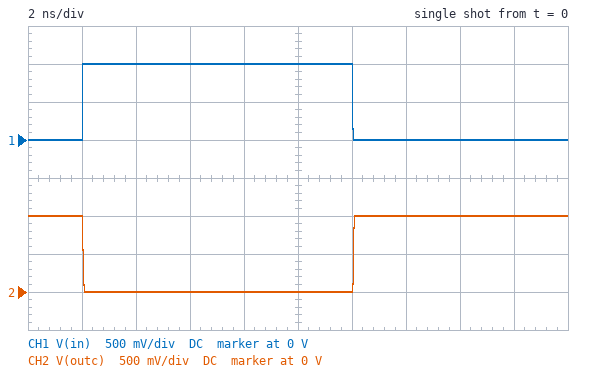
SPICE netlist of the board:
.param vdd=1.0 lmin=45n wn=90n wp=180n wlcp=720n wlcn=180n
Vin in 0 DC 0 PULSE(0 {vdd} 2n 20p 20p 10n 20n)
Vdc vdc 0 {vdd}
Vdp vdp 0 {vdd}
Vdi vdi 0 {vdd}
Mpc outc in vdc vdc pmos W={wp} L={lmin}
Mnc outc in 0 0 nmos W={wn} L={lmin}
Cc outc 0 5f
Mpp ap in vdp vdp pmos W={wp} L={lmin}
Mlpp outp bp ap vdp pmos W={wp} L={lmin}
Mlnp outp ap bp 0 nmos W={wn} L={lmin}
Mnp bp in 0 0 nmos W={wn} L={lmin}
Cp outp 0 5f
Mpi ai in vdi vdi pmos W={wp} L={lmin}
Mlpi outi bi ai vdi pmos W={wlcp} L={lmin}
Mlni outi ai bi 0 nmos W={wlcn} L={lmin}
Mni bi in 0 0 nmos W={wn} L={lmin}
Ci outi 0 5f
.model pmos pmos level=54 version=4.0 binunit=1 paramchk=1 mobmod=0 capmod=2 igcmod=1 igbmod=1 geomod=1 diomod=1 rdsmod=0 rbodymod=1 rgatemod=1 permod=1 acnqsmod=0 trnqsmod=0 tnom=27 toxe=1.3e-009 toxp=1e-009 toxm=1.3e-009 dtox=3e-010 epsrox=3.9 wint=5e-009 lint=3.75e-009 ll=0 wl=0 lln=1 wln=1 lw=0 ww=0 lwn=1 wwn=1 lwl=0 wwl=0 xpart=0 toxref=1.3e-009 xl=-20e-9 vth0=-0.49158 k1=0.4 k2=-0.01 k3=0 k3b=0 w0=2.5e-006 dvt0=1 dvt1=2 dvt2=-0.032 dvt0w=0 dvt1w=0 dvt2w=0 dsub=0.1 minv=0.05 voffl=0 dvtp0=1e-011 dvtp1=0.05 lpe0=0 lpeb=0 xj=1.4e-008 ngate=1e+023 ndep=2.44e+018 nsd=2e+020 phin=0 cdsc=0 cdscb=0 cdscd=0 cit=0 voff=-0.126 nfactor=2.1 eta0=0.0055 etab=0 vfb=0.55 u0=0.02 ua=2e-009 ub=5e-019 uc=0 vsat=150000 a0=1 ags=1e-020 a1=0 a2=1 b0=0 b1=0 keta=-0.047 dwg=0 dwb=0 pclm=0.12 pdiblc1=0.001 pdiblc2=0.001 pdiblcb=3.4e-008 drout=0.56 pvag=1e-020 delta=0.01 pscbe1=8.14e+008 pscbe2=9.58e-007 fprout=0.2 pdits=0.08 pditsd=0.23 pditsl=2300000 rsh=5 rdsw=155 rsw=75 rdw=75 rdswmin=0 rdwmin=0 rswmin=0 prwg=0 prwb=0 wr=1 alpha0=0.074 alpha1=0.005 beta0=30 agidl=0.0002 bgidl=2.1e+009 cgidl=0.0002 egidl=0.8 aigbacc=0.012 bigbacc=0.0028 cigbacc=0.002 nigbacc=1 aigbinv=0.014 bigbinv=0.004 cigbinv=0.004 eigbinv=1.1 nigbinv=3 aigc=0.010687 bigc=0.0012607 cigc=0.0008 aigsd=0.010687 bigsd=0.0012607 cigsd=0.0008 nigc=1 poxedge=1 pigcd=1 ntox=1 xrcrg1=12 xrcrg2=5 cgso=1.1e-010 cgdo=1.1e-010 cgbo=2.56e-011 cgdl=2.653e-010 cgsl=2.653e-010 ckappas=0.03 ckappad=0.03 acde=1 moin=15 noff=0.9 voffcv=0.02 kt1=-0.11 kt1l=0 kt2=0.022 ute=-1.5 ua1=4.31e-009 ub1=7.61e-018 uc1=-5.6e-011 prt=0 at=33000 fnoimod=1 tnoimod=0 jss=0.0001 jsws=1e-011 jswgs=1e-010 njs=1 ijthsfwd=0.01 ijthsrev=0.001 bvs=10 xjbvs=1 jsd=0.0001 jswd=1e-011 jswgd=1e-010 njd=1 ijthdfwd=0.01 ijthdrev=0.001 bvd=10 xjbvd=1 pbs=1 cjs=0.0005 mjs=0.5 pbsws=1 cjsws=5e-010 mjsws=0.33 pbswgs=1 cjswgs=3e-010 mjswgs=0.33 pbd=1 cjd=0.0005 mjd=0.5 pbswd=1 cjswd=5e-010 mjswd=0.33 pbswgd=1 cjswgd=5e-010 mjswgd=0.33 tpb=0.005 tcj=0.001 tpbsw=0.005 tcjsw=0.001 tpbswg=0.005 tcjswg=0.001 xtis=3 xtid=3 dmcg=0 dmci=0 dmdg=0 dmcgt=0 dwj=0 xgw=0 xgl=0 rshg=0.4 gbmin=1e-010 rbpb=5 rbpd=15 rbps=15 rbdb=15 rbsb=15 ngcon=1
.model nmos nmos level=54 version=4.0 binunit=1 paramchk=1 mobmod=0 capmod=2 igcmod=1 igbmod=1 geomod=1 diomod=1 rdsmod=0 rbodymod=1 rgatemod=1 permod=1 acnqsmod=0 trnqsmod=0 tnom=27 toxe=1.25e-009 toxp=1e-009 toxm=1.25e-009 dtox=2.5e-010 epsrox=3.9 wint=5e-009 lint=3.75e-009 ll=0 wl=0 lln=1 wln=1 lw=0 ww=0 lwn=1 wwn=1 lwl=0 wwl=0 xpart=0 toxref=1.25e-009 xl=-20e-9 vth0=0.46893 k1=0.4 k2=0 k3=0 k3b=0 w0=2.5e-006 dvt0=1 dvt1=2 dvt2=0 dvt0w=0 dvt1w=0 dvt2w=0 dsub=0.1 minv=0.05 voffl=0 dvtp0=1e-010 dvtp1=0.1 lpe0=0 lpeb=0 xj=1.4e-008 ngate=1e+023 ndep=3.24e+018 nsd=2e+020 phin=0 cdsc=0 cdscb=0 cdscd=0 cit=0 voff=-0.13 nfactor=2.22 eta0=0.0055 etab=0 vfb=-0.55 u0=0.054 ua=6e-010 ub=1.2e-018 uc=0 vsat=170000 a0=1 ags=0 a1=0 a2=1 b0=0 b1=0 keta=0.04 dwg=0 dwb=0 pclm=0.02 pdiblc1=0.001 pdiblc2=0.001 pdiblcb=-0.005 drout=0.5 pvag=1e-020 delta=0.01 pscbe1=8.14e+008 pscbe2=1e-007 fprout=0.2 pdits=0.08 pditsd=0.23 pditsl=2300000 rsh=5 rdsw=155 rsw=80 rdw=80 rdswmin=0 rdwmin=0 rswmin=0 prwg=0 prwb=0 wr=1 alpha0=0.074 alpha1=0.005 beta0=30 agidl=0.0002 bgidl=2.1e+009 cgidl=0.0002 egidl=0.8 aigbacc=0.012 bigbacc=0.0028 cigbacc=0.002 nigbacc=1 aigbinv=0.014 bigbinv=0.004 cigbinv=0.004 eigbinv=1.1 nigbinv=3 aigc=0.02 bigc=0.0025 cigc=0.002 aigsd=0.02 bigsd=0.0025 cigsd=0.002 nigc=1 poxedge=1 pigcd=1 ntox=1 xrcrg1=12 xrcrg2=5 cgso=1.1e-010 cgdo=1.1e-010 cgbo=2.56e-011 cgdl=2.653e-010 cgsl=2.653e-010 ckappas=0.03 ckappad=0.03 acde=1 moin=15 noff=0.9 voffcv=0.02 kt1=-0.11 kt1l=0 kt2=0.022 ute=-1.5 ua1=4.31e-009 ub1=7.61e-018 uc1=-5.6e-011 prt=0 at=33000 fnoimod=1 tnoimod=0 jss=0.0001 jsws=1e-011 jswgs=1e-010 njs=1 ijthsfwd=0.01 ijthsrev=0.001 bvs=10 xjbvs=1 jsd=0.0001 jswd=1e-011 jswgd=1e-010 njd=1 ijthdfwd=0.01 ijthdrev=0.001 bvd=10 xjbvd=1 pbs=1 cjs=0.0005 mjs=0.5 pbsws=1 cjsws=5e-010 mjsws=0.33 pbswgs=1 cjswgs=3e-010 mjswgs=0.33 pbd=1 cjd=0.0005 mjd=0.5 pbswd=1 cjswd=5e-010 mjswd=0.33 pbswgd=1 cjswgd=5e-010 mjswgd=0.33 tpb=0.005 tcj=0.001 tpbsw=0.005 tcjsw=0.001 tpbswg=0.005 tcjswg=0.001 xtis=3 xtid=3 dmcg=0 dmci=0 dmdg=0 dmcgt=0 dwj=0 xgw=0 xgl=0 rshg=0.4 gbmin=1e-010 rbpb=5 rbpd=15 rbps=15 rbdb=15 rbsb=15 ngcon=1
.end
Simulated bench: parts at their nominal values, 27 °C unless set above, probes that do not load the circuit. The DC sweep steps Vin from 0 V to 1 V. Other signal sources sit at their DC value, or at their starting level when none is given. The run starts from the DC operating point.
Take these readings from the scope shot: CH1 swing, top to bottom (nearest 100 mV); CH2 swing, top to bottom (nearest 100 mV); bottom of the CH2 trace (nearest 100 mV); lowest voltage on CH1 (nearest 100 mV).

1.0 V
1.0 V
0 V
0 V
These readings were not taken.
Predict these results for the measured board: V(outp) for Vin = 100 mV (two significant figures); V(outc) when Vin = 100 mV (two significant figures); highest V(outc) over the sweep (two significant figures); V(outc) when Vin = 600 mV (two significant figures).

990 mV
1.0 V
1.0 V
43 mV
